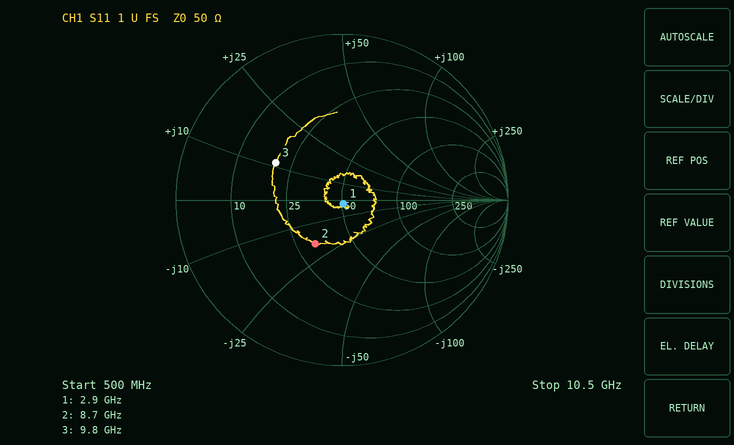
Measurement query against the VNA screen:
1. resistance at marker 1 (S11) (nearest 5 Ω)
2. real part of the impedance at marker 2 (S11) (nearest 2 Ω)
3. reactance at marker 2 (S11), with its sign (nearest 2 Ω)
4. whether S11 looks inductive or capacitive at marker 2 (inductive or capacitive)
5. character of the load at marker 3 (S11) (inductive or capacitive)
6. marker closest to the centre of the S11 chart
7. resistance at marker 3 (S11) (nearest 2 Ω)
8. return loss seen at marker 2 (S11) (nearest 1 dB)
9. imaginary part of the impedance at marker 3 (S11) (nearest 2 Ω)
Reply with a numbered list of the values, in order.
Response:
1. 50 Ω
2. 32 Ω
3. -18 Ω
4. capacitive
5. inductive
6. marker 1
7. 20 Ω
8. 10 dB
9. +12 Ω
